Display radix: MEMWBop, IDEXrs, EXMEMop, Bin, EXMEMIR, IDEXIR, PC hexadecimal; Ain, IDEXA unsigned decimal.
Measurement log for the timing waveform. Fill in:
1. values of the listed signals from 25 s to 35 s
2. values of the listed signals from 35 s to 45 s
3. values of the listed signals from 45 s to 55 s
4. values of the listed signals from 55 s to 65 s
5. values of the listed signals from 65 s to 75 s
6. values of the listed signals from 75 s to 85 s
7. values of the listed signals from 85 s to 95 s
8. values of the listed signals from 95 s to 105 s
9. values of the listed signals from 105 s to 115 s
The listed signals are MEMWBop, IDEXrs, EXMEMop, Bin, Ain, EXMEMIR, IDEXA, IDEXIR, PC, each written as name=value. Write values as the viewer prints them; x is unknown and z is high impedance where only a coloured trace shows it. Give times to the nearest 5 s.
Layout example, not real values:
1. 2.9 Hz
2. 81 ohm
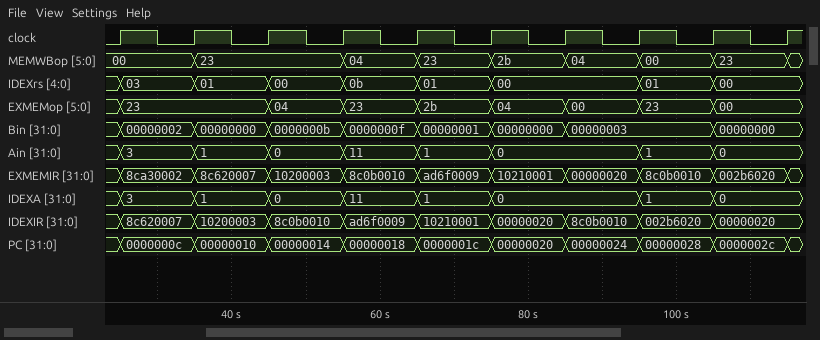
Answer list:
1. MEMWBop=00, IDEXrs=03, EXMEMop=23, Bin=00000002, Ain=3, EXMEMIR=8ca30002, IDEXA=3, IDEXIR=8c620007, PC=0000000c
2. MEMWBop=23, IDEXrs=01, EXMEMop=23, Bin=00000000, Ain=1, EXMEMIR=8c620007, IDEXA=1, IDEXIR=10200003, PC=00000010
3. MEMWBop=23, IDEXrs=00, EXMEMop=04, Bin=0000000b, Ain=0, EXMEMIR=10200003, IDEXA=0, IDEXIR=8c0b0010, PC=00000014
4. MEMWBop=04, IDEXrs=0b, EXMEMop=23, Bin=0000000f, Ain=11, EXMEMIR=8c0b0010, IDEXA=11, IDEXIR=ad6f0009, PC=00000018
5. MEMWBop=23, IDEXrs=01, EXMEMop=2b, Bin=00000001, Ain=1, EXMEMIR=ad6f0009, IDEXA=1, IDEXIR=10210001, PC=0000001c
6. MEMWBop=2b, IDEXrs=00, EXMEMop=04, Bin=00000000, Ain=0, EXMEMIR=10210001, IDEXA=0, IDEXIR=00000020, PC=00000020
7. MEMWBop=04, IDEXrs=00, EXMEMop=00, Bin=00000003, Ain=0, EXMEMIR=00000020, IDEXA=0, IDEXIR=8c0b0010, PC=00000024
8. MEMWBop=00, IDEXrs=01, EXMEMop=23, Bin=00000003, Ain=1, EXMEMIR=8c0b0010, IDEXA=1, IDEXIR=002b6020, PC=00000028
9. MEMWBop=23, IDEXrs=00, EXMEMop=00, Bin=00000000, Ain=0, EXMEMIR=002b6020, IDEXA=0, IDEXIR=00000020, PC=0000002c
